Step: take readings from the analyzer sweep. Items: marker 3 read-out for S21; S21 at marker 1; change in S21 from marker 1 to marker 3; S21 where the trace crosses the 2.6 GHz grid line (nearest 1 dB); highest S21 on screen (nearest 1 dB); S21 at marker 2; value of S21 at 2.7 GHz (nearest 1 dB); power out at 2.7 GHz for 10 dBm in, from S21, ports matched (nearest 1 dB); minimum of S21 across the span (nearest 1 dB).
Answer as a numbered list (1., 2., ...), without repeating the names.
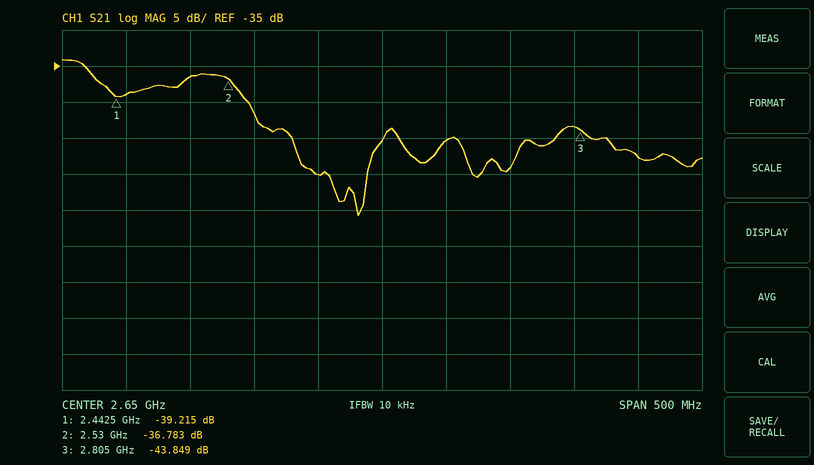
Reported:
1. -43.849 dB
2. -39.215 dB
3. -4.634 dB
4. -50 dB
5. -34 dB
6. -36.783 dB
7. -45 dB
8. -35 dBm
9. -56 dB
